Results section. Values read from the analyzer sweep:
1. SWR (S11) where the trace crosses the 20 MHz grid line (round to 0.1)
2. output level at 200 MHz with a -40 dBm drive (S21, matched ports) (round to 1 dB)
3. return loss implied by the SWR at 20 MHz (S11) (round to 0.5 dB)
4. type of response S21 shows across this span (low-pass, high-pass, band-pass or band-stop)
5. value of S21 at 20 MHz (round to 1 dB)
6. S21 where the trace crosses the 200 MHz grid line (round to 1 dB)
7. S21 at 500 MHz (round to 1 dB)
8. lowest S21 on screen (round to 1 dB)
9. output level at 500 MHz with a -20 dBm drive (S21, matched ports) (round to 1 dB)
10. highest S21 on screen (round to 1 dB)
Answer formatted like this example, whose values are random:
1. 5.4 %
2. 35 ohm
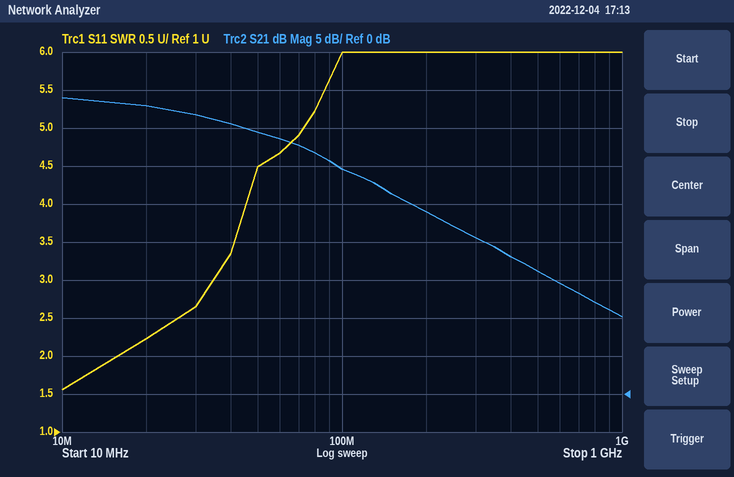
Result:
1. 2.2
2. -16 dBm
3. 8.5 dB
4. low-pass
5. 38 dB
6. 24 dB
7. 16 dB
8. 10 dB
9. -4 dBm
10. 39 dB
